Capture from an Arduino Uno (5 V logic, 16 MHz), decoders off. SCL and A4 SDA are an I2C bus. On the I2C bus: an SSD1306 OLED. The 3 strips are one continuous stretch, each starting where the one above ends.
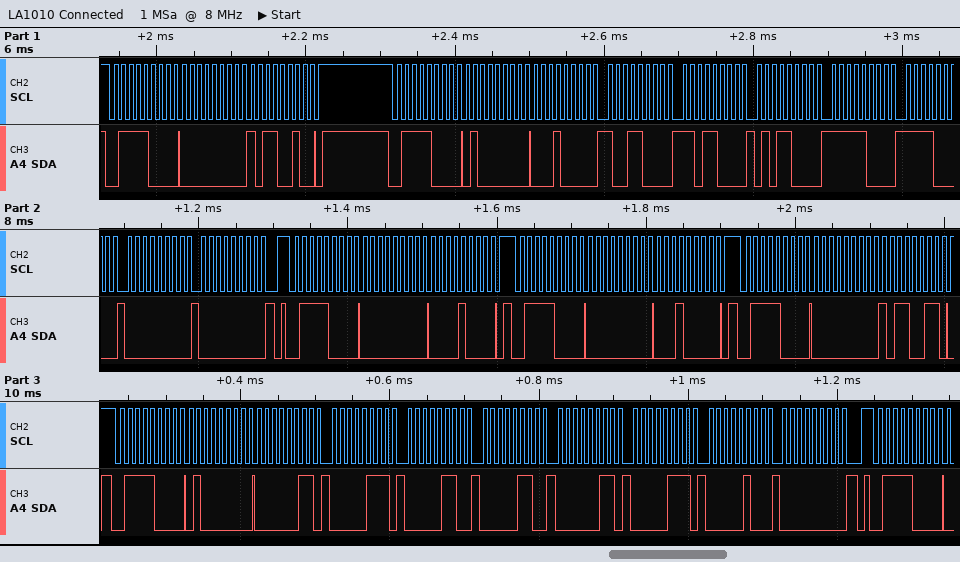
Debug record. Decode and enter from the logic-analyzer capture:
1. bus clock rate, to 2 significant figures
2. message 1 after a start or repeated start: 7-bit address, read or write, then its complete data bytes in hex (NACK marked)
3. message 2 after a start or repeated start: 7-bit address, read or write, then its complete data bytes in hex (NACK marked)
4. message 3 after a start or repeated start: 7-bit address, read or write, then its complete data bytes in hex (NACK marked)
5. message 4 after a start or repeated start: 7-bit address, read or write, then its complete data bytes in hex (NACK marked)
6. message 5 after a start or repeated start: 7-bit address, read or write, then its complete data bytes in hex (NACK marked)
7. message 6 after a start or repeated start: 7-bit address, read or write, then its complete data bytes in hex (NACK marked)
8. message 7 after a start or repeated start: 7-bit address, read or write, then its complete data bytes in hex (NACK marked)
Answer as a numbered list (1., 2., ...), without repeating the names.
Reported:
1. 100 kHz
2. 0x3C write: 00 B2
3. 0x3C write: 40 10 98 D8 58 F8 F0 00 00
4. 0x3C write: 00 08
5. 0x3C write: 00 10
6. 0x3C write: 00 B3
7. 0x3C write: 40 03 07 06 06 03 07 04 00
8. 0x3C write
